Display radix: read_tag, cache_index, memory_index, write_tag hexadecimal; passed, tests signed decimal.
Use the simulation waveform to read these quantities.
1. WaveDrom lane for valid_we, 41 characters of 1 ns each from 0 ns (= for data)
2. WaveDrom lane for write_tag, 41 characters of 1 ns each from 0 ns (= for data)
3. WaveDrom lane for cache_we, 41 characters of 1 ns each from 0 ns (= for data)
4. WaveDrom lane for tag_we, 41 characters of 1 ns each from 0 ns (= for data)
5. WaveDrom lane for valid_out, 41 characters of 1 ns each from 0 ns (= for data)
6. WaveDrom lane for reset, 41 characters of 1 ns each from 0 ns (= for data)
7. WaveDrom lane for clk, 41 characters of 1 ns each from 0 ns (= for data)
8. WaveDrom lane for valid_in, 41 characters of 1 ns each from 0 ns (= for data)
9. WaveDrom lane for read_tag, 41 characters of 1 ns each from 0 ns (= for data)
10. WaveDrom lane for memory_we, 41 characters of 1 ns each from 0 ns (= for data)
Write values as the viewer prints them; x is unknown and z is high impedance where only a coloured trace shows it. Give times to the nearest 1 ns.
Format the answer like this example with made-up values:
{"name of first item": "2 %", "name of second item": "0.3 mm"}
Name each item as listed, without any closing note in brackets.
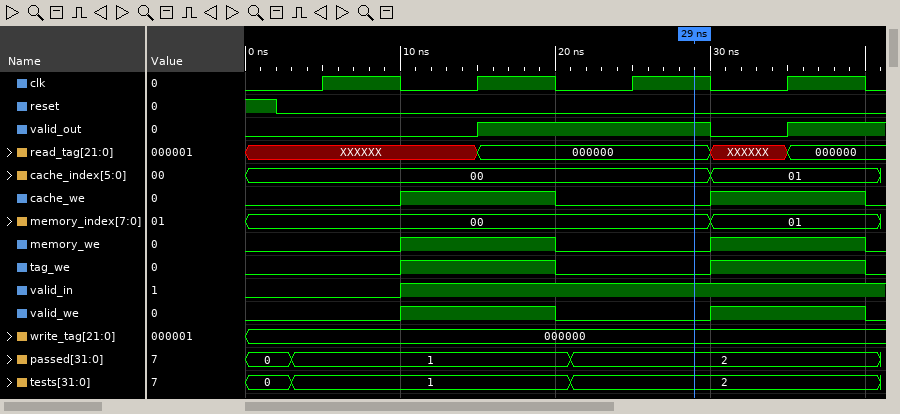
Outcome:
{"WaveDrom lane for valid_we, 41 characters of 1 ns each from 0 ns": "{name: 'valid_we', wave: '0.........1.........0.........1.........0'}", "WaveDrom lane for write_tag, 41 characters of 1 ns each from 0 ns": "{name: 'write_tag', wave: '=........................................', data: '000000'}", "WaveDrom lane for cache_we, 41 characters of 1 ns each from 0 ns": "{name: 'cache_we', wave: '0.........1.........0.........1.........0'}", "WaveDrom lane for tag_we, 41 characters of 1 ns each from 0 ns": "{name: 'tag_we', wave: '0.........1.........0.........1.........0'}", "WaveDrom lane for valid_out, 41 characters of 1 ns each from 0 ns": "{name: 'valid_out', wave: '0..............1..............0....1.....'}", "WaveDrom lane for reset, 41 characters of 1 ns each from 0 ns": "{name: 'reset', wave: '1.0......................................'}", "WaveDrom lane for clk, 41 characters of 1 ns each from 0 ns": "{name: 'clk', wave: '0....1....0....1....0....1....0....1....0'}", "WaveDrom lane for valid_in, 41 characters of 1 ns each from 0 ns": "{name: 'valid_in', wave: '0.........1..............................'}", "WaveDrom lane for read_tag, 41 characters of 1 ns each from 0 ns": "{name: 'read_tag', wave: 'x..............=..............x....=.....', data: '000000 000000'}", "WaveDrom lane for memory_we, 41 characters of 1 ns each from 0 ns": "{name: 'memory_we', wave: '0.........1.........0.........1.........0'}"}
